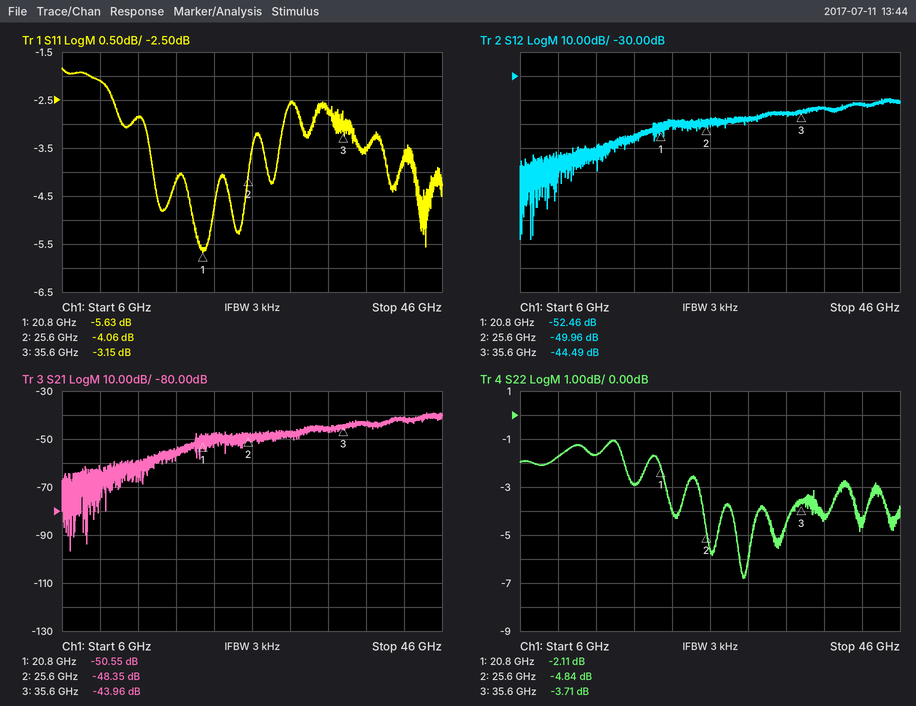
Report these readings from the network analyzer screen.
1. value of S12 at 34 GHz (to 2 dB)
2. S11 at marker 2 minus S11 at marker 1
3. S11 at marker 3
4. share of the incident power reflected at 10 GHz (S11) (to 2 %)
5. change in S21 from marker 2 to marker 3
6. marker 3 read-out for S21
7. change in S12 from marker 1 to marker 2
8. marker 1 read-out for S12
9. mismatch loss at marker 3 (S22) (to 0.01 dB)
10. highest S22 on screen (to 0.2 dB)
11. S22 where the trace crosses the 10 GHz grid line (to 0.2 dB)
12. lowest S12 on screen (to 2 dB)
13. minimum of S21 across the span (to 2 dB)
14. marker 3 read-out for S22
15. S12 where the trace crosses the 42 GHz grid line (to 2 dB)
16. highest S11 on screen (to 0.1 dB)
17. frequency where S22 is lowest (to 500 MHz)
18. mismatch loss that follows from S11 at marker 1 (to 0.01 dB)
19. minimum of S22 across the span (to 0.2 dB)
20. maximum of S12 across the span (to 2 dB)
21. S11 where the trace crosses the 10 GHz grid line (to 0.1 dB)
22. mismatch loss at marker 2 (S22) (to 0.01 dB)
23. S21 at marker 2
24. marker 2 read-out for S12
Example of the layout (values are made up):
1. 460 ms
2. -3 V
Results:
1. -46 dB
2. 1.57 dB
3. -3.15 dB
4. 62 %
5. 4.39 dB
6. -43.96 dB
7. 2.50 dB
8. -52.46 dB
9. 2.41 dB
10. -1.0 dB
11. -1.8 dB
12. -98 dB
13. -96 dB
14. -3.71 dB
15. -42 dB
16. -1.8 dB
17. 29.5 GHz
18. 1.39 dB
19. -6.8 dB
20. -40 dB
21. -2.1 dB
22. 1.73 dB
23. -48.35 dB
24. -49.96 dB
